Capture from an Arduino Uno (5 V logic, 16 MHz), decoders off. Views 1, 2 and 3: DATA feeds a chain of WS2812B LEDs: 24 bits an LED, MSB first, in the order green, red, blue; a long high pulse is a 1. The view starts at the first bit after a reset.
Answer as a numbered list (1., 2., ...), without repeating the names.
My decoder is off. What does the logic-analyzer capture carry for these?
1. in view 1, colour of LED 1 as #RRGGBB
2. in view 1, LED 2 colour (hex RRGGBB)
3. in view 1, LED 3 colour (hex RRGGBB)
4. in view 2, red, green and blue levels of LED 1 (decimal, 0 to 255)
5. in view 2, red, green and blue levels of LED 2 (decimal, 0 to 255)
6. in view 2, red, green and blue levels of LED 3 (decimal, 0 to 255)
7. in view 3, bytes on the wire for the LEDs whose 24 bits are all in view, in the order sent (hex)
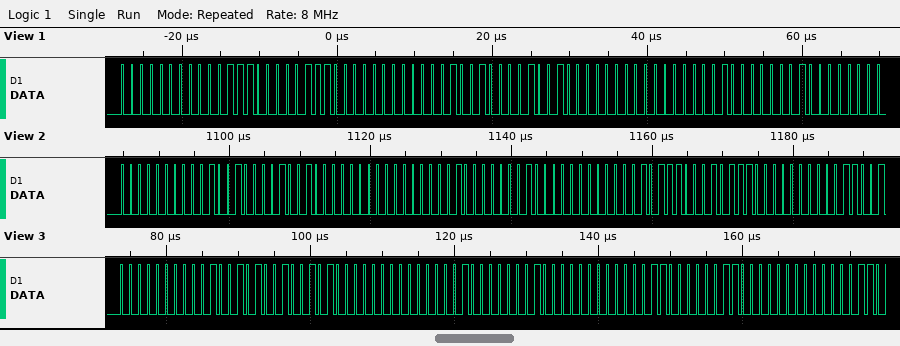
1. #1C001C
2. #240024
3. #020002
4. 36, 0, 36
5. 2, 0, 2
6. 23, 0, 23
7. 00 25 25 00 02 02 00 18 18
